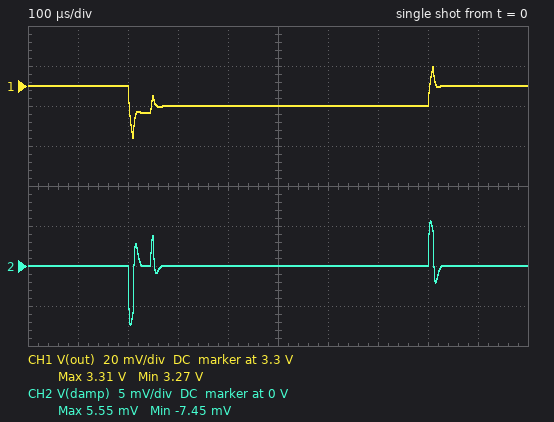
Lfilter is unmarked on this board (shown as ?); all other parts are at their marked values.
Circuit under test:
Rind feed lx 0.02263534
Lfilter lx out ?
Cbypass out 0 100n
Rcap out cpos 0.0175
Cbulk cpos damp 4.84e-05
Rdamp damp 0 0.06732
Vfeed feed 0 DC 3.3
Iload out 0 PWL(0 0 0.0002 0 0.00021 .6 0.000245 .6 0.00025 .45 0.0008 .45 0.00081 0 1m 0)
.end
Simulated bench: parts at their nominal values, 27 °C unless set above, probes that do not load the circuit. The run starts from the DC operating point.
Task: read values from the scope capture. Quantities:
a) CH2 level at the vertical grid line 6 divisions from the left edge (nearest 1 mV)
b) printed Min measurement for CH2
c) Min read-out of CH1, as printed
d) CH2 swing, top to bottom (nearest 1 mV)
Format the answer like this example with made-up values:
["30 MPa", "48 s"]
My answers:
["0 V", "-7.45 mV", "3.27 V", "13 mV"]
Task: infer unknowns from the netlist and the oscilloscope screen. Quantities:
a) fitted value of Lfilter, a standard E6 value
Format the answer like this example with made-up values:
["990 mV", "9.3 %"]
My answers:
["220 nH"]
